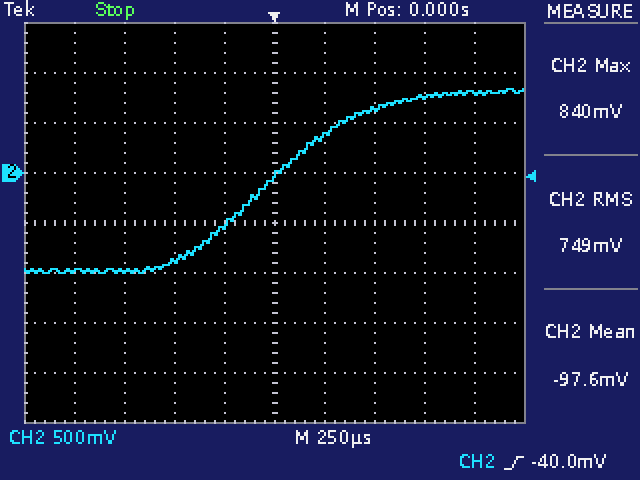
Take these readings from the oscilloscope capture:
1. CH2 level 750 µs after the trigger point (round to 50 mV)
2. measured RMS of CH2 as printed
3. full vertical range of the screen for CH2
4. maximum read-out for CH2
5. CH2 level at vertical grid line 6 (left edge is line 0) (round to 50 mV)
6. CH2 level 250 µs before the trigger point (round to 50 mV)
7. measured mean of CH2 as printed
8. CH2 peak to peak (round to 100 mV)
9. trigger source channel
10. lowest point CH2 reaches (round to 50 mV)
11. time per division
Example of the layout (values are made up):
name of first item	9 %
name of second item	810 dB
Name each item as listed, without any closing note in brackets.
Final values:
CH2 level 750 µs after the trigger point	750 mV
measured RMS of CH2 as printed	749 mV
full vertical range of the screen for CH2	4 V
maximum read-out for CH2	840 mV
CH2 level at vertical grid line 6 (left edge is line 0)	350 mV
CH2 level 250 µs before the trigger point	-500 mV
measured mean of CH2 as printed	-97.6 mV
CH2 peak to peak	1.80 V
trigger source channel	CH2
lowest point CH2 reaches	-1.00 V
time per division	250 µs
